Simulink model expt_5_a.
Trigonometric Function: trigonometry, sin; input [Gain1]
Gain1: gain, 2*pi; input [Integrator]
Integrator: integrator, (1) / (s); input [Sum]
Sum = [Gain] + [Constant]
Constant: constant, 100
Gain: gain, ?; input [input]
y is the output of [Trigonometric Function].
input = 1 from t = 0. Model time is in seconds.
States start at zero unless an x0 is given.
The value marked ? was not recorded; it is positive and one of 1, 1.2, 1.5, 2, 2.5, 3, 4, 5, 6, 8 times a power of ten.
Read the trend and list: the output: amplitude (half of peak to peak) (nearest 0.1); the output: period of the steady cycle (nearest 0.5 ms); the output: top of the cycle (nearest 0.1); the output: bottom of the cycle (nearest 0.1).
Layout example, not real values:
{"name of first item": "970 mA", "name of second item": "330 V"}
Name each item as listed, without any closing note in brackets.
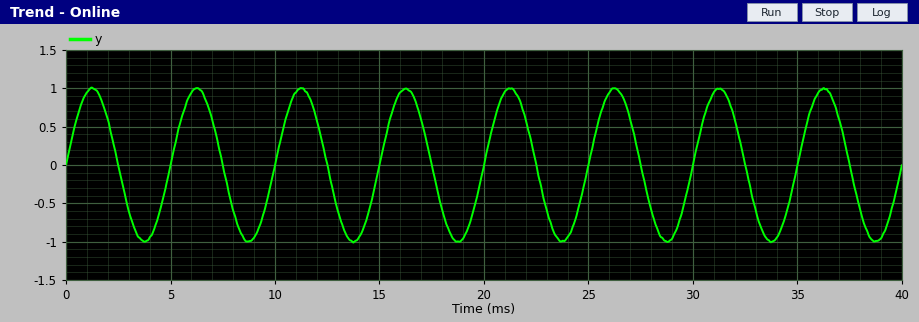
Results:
{"the output: amplitude (half of peak to peak)": "1.0", "the output: period of the steady cycle": "5.0 ms", "the output: top of the cycle": "1.0", "the output: bottom of the cycle": "-1.0"}
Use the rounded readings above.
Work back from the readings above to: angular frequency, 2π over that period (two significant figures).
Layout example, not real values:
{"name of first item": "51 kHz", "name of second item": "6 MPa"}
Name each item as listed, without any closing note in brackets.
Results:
{"angular frequency, 2π over that period": "1.3 rad/ms"}
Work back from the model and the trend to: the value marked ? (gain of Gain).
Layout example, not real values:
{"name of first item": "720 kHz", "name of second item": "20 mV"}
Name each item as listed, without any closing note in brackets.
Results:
{"the value marked ?": "100"}
